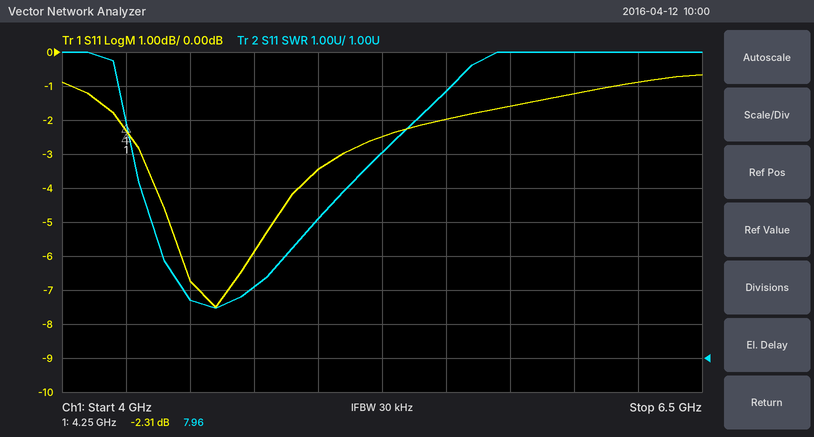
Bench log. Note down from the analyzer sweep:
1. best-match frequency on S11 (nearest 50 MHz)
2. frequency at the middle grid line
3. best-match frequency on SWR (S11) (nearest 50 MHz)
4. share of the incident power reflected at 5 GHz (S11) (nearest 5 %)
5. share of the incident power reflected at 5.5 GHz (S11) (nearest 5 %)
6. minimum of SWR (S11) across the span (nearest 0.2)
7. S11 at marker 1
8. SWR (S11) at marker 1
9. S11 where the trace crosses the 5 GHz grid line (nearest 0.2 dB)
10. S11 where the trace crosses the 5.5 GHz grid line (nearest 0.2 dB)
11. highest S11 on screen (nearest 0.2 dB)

4.60 GHz
5.25 GHz
4.60 GHz
45 %
65 %
2.4
-2.31 dB
7.96
-3.4 dB
-2.0 dB
-0.6 dB
